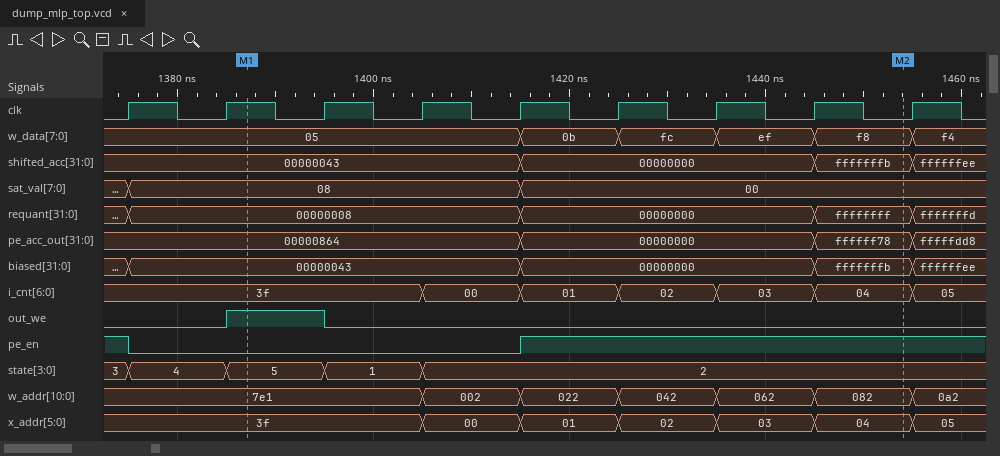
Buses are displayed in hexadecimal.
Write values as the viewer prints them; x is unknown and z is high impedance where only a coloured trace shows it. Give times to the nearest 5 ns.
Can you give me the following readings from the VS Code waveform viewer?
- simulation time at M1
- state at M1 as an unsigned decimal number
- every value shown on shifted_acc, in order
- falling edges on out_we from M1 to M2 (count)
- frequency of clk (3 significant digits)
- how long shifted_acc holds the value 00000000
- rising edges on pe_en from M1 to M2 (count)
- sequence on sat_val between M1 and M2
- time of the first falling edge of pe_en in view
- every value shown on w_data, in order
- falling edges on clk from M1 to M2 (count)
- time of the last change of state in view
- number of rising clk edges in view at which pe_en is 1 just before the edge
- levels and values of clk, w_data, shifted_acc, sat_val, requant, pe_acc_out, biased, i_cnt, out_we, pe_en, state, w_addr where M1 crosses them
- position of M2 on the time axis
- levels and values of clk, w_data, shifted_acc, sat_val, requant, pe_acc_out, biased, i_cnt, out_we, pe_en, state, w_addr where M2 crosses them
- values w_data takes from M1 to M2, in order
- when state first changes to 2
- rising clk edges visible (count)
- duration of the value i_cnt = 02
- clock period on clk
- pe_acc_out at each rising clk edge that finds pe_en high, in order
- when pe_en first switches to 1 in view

1385 ns
5
00000043, 00000000, fffffffb, ffffffee
1
100 MHz
30 ns
1
08, 00
1375 ns
05, 0b, fc, ef, f8, f4
7
1405 ns
5
clk=1, w_data=05, shifted_acc=00000043, sat_val=08, requant=00000008, pe_acc_out=00000864, biased=00000043, i_cnt=3f, out_we=1, pe_en=0, state=5, w_addr=7e1
1455 ns
clk=0, w_data=f8, shifted_acc=fffffffb, sat_val=00, requant=ffffffff, pe_acc_out=ffffff78, biased=fffffffb, i_cnt=04, out_we=0, pe_en=1, state=2, w_addr=082
05, 0b, fc, ef, f8
1405 ns
9
10 ns
10 ns
00000864, 00000000, 00000000, 00000000, ffffff78
1415 ns
